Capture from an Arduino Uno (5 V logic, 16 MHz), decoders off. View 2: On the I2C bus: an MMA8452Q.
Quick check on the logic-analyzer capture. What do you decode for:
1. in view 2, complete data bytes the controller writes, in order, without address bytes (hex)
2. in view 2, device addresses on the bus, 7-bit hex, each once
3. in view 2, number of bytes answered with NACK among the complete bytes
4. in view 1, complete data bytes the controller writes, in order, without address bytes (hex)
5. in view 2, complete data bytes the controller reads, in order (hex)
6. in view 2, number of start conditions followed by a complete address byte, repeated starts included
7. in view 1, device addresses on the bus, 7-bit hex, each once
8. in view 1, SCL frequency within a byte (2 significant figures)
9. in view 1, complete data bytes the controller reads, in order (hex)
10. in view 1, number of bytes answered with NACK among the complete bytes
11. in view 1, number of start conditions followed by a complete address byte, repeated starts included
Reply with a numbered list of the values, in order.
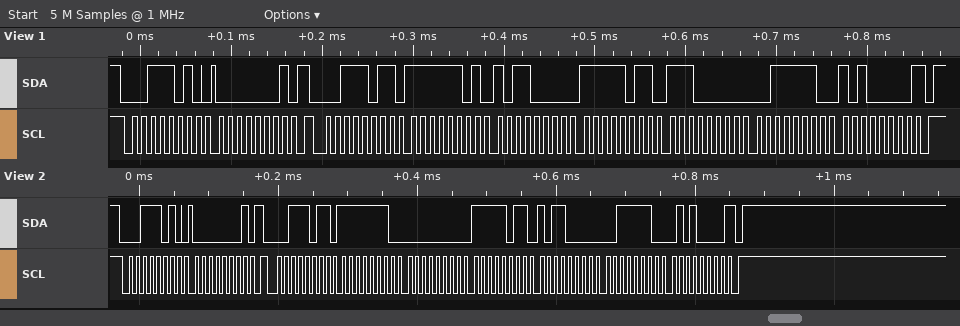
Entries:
1. 01
2. 0x1D
3. 1
4. 01
5. FE 00 FB B0 3E 50
6. 2
7. 0x1D
8. 100 kHz
9. FD B0 FB E0 3E A0
10. 1
11. 2
